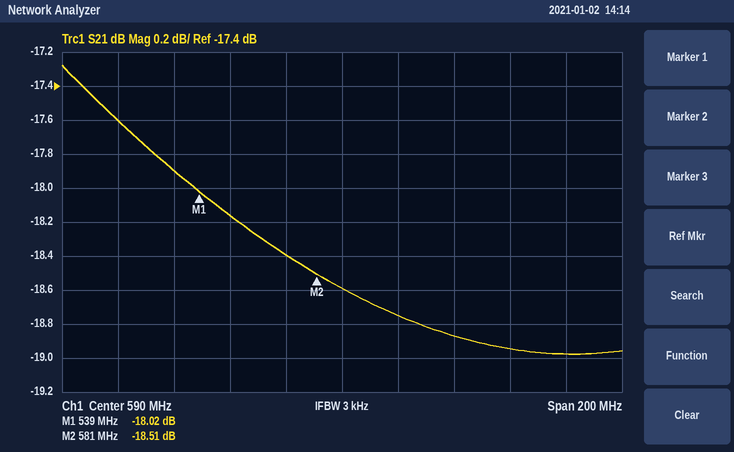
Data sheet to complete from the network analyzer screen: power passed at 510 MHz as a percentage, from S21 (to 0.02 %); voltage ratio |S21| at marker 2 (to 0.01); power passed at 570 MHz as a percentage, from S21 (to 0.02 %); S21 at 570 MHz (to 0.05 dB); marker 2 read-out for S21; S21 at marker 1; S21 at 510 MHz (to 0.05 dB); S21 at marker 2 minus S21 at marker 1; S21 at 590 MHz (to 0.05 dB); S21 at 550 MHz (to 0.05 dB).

1.74 %
0.12
1.44 %
-18.40 dB
-18.51 dB
-18.02 dB
-17.60 dB
-0.49 dB
-18.60 dB
-18.15 dB
